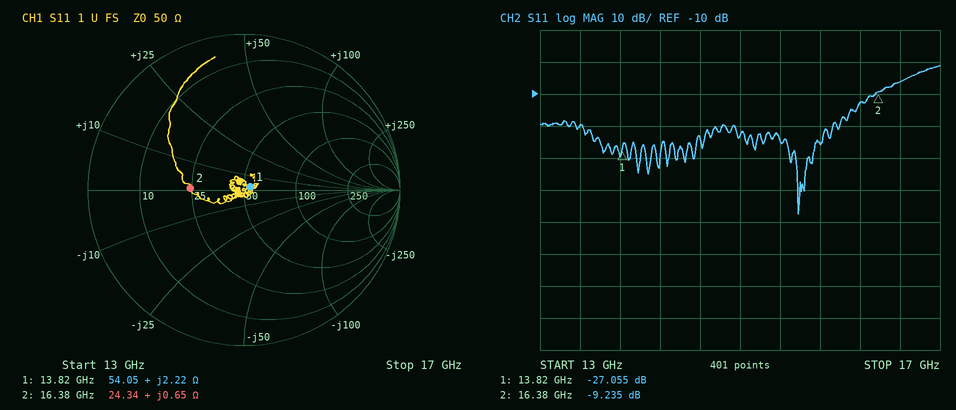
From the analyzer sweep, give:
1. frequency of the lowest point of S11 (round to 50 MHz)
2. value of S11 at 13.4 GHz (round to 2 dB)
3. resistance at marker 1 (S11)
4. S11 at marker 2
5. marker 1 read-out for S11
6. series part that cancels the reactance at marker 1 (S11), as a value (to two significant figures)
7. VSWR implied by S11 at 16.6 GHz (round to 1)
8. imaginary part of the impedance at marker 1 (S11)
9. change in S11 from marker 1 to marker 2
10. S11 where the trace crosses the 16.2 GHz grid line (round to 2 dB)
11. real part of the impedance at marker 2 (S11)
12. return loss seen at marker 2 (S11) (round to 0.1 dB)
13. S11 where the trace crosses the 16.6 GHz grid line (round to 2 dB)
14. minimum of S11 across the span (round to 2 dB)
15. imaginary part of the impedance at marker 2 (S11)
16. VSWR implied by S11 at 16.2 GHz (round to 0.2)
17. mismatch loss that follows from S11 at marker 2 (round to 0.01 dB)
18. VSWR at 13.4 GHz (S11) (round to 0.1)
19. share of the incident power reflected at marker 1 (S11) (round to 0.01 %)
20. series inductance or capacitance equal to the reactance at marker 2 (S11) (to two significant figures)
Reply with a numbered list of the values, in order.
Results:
1. 15.60 GHz
2. -20 dB
3. 54.05 Ω
4. -9.235 dB
5. -27.055 dB
6. 5.2 pF
7. 3
8. +2.22 Ω
9. 17.820 dB
10. -12 dB
11. 24.34 Ω
12. 9.2 dB
13. -6 dB
14. -48 dB
15. +0.65 Ω
16. 1.6
17. 0.55 dB
18. 1.2
19. 0.20 %
20. 6.3 pH
